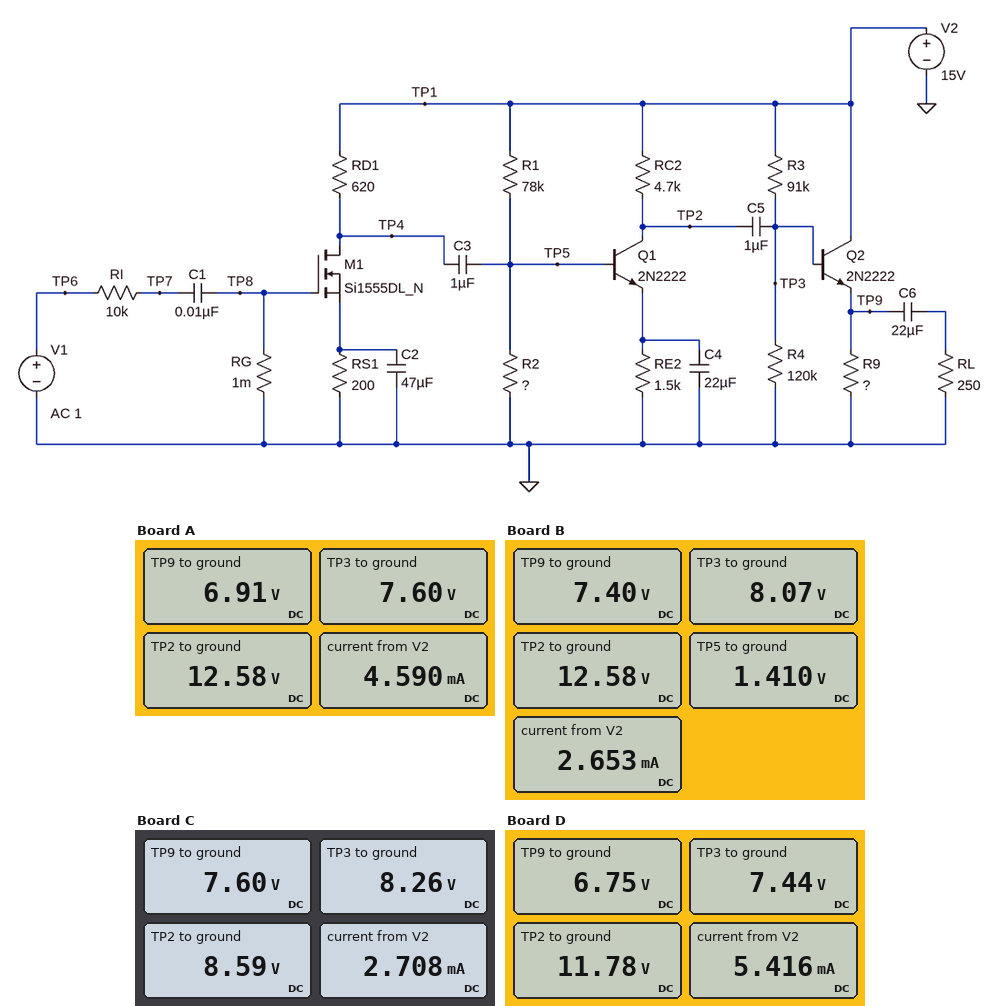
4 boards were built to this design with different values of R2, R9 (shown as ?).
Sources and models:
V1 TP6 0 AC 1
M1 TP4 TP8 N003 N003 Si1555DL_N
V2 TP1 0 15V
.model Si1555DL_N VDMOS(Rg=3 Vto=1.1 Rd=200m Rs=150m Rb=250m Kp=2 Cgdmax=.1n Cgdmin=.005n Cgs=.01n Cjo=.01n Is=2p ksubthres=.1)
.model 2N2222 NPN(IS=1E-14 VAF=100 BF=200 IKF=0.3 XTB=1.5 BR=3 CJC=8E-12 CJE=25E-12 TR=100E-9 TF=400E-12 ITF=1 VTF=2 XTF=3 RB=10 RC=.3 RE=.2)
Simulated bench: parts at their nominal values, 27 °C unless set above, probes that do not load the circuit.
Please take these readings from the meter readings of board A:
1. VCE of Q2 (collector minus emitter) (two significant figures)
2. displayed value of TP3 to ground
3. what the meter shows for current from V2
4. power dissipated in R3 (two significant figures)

8.1 V
7.60 V
4.590 mA
600 µW
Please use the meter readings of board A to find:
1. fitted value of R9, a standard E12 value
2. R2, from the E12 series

1.8 kΩ
8.2 kΩ
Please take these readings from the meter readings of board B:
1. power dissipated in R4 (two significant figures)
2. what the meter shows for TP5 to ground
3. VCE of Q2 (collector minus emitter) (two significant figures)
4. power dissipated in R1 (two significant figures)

540 µW
1.410 V
7.6 V
2.4 mW
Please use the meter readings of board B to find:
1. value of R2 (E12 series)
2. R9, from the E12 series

8.2 kΩ
3.9 kΩ
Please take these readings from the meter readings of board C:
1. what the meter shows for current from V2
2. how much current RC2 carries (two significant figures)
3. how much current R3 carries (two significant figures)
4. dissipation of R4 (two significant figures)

2.708 mA
1.4 mA
74 µA
570 µW
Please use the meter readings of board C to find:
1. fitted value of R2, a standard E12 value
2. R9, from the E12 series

18 kΩ
6.8 kΩ
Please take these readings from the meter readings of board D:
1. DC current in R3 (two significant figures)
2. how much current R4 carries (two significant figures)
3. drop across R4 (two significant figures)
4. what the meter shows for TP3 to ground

83 µA
62 µA
7.4 V
7.44 V
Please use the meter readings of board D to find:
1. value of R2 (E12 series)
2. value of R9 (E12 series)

10 kΩ
1.5 kΩ
